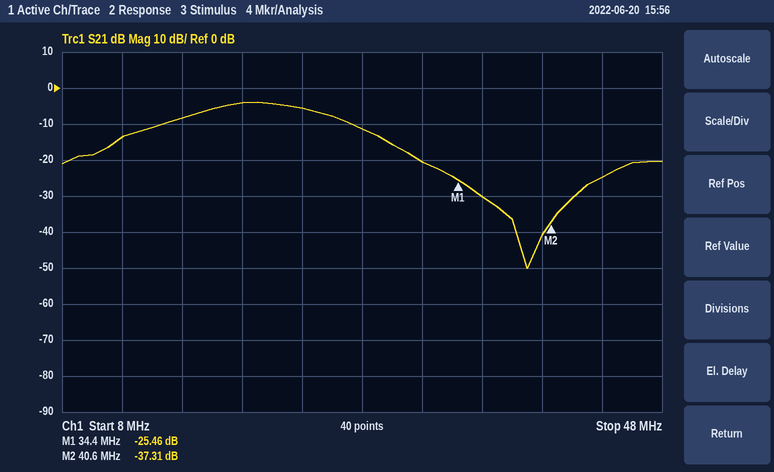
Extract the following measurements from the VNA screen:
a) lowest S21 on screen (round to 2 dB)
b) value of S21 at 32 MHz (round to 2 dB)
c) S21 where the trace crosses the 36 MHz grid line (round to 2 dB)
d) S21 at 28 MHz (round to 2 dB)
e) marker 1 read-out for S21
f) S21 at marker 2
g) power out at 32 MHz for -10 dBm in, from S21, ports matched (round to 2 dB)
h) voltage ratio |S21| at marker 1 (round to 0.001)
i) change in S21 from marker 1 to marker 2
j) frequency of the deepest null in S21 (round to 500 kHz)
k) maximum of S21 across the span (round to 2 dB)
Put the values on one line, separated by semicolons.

-50 dB; -20 dB; -30 dB; -12 dB; -25.46 dB; -37.31 dB; -30 dBm; 0.053; -11.85 dB; 39.0 MHz; -4 dB
